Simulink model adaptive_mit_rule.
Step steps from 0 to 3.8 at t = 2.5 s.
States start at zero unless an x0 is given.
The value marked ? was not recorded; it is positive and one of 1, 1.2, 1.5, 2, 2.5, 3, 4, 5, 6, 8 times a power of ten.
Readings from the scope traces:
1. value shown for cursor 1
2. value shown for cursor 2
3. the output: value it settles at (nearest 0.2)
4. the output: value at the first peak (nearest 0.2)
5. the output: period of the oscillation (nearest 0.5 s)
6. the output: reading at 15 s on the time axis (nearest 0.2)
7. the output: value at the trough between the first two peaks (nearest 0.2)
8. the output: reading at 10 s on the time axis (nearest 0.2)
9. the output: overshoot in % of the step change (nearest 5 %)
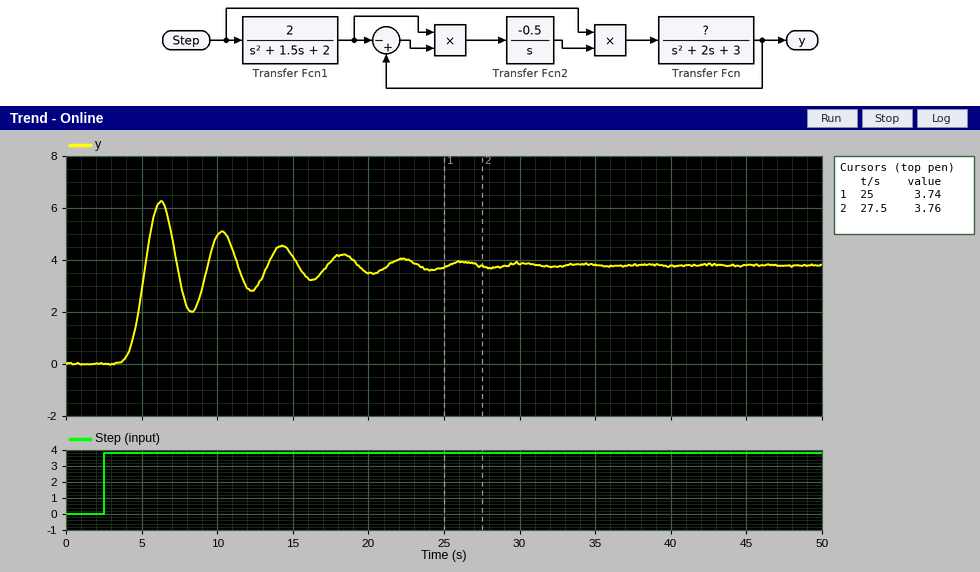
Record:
3.74
3.76
3.8
6.2
4.0 s
4.2
2.0
5.0
65 %
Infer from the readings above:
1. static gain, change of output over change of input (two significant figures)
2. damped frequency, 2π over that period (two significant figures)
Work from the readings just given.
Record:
1.0
1.6 rad/s
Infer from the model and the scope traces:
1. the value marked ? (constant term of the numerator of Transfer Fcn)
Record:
0.6
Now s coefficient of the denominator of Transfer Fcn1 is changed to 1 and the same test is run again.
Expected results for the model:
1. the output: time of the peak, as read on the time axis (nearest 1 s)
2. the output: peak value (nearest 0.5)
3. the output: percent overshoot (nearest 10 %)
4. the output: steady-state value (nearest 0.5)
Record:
6 s
7.5
100 %
4.0
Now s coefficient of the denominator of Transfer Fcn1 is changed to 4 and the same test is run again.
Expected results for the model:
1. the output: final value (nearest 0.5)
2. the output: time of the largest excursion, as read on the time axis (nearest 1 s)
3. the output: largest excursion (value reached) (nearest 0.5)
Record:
4.0
11 s
4.0
